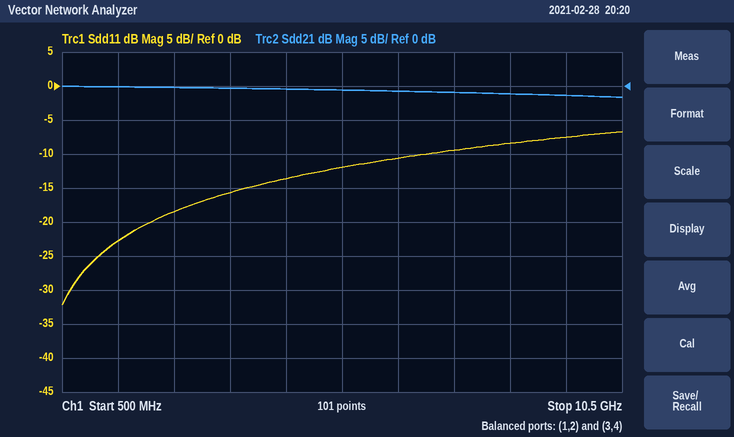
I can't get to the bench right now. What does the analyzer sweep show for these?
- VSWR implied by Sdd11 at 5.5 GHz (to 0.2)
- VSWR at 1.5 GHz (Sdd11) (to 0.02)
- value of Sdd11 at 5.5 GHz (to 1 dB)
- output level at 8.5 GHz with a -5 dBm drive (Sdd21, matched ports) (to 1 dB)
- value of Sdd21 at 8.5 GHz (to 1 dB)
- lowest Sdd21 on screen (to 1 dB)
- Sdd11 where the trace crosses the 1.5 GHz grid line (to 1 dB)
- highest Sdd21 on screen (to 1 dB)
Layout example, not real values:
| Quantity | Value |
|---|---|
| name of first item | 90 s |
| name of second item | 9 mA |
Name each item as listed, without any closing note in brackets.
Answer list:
| Quantity | Value |
|---|---|
| VSWR implied by Sdd11 at 5.5 GHz | 1.6 |
| VSWR at 1.5 GHz (Sdd11) | 1.16 |
| value of Sdd11 at 5.5 GHz | -12 dB |
| output level at 8.5 GHz with a -5 dBm drive (Sdd21, matched ports) | -6 dBm |
| value of Sdd21 at 8.5 GHz | -1 dB |
| lowest Sdd21 on screen | -2 dB |
| Sdd11 where the trace crosses the 1.5 GHz grid line | -23 dB |
| highest Sdd21 on screen | 0 dB |
